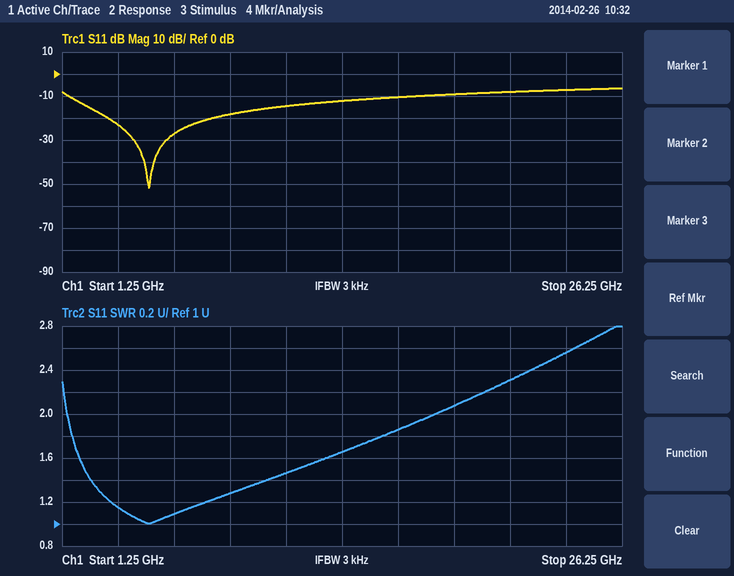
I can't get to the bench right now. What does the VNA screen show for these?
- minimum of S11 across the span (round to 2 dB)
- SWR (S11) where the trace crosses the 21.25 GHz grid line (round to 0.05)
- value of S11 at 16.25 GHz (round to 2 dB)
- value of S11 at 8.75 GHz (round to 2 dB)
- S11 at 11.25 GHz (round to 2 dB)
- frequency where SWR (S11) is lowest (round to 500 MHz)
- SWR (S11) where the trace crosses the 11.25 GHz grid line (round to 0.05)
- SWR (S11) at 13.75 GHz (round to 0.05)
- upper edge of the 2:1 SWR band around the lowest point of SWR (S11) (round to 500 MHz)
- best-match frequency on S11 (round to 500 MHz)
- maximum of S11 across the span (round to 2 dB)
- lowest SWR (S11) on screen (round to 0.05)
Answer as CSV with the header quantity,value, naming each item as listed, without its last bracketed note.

quantity,value
minimum of S11 across the span,-52 dB
SWR (S11) where the trace crosses the 21.25 GHz grid line,2.30
value of S11 at 16.25 GHz,-10 dB
value of S11 at 8.75 GHz,-18 dB
S11 at 11.25 GHz,-14 dB
frequency where SWR (S11) is lowest,5.0 GHz
SWR (S11) where the trace crosses the 11.25 GHz grid line,1.45
SWR (S11) at 13.75 GHz,1.65
upper edge of the 2:1 SWR band around the lowest point of SWR (S11),18.0 GHz
best-match frequency on S11,5.0 GHz
maximum of S11 across the span,-6 dB
lowest SWR (S11) on screen,1.00
